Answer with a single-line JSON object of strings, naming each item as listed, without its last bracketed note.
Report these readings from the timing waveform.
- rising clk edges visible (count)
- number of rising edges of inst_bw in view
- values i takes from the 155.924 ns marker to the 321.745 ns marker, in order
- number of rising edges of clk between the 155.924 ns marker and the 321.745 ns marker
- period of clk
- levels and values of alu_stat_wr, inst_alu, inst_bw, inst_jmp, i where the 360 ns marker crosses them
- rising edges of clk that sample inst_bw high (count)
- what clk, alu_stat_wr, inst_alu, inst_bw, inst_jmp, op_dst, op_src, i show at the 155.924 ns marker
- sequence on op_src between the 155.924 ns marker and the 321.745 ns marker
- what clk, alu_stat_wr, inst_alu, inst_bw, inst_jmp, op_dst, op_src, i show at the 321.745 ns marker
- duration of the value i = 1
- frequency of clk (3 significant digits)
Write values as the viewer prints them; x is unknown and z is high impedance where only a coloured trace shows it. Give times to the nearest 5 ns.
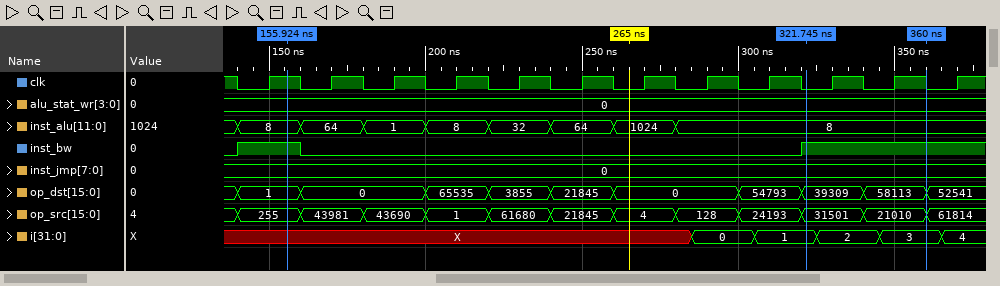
{"rising clk edges visible": "12", "number of rising edges of inst_bw in view": "2", "values i takes from the 155.924 ns marker to the 321.745 ns marker, in order": "X, 0, 1", "number of rising edges of clk between the 155.924 ns marker and the 321.745 ns marker": "8", "period of clk": "20 ns", "levels and values of alu_stat_wr, inst_alu, inst_bw, inst_jmp, i where the 360 ns marker crosses them": "alu_stat_wr=0, inst_alu=8, inst_bw=1, inst_jmp=0, i=3", "rising edges of clk that sample inst_bw high": "4", "what clk, alu_stat_wr, inst_alu, inst_bw, inst_jmp, op_dst, op_src, i show at the 155.924 ns marker": "clk=1, alu_stat_wr=0, inst_alu=8, inst_bw=1, inst_jmp=0, op_dst=1, op_src=255, i=X", "sequence on op_src between the 155.924 ns marker and the 321.745 ns marker": "255, 43981, 43690, 1, 61680, 21845, 4, 128, 24193, 31501", "what clk, alu_stat_wr, inst_alu, inst_bw, inst_jmp, op_dst, op_src, i show at the 321.745 ns marker": "clk=0, alu_stat_wr=0, inst_alu=8, inst_bw=1, inst_jmp=0, op_dst=39309, op_src=31501, i=1", "duration of the value i = 1": "20 ns", "frequency of clk": "50.0 MHz"}
